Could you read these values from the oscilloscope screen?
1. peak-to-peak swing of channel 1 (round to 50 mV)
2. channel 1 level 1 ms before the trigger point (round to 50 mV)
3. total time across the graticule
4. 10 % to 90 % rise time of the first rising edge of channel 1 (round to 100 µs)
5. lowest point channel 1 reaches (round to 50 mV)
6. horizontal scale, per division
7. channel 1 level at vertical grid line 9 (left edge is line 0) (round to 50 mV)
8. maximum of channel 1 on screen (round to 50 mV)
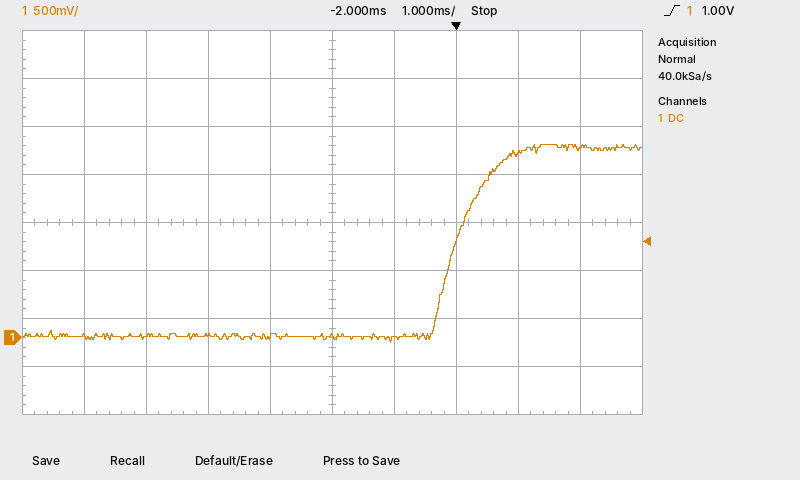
2.05 V
0 mV
10 ms
1.0 ms
-50 mV
1 ms
2.00 V
2.00 V
